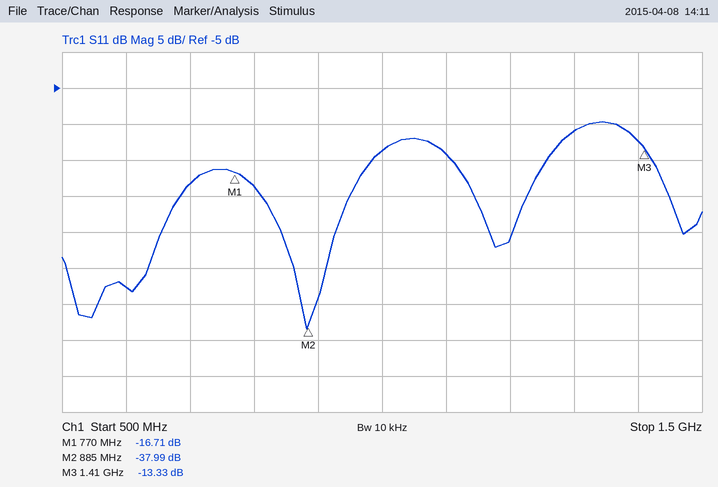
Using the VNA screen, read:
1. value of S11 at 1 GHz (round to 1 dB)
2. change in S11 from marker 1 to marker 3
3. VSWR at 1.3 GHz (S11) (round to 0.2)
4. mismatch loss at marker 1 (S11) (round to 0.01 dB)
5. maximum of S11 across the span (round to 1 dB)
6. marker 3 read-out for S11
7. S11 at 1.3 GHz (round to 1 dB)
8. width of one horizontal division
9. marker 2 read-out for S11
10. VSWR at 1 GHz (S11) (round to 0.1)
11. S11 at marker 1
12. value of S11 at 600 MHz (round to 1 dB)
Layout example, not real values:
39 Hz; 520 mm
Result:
-14 dB; 3.38 dB; 1.8; 0.09 dB; -10 dB; -13.33 dB; -11 dB; 100 MHz; -37.99 dB; 1.5; -16.71 dB; -33 dB
